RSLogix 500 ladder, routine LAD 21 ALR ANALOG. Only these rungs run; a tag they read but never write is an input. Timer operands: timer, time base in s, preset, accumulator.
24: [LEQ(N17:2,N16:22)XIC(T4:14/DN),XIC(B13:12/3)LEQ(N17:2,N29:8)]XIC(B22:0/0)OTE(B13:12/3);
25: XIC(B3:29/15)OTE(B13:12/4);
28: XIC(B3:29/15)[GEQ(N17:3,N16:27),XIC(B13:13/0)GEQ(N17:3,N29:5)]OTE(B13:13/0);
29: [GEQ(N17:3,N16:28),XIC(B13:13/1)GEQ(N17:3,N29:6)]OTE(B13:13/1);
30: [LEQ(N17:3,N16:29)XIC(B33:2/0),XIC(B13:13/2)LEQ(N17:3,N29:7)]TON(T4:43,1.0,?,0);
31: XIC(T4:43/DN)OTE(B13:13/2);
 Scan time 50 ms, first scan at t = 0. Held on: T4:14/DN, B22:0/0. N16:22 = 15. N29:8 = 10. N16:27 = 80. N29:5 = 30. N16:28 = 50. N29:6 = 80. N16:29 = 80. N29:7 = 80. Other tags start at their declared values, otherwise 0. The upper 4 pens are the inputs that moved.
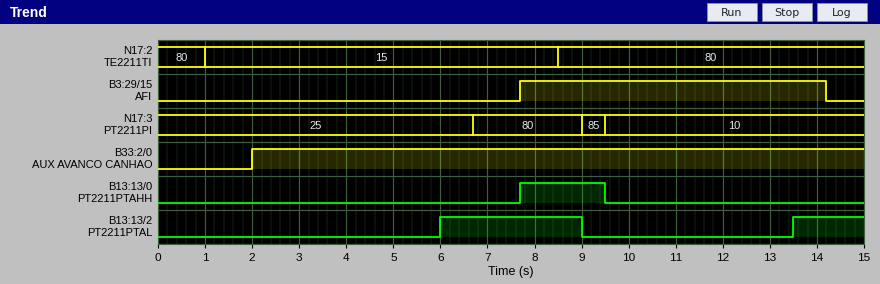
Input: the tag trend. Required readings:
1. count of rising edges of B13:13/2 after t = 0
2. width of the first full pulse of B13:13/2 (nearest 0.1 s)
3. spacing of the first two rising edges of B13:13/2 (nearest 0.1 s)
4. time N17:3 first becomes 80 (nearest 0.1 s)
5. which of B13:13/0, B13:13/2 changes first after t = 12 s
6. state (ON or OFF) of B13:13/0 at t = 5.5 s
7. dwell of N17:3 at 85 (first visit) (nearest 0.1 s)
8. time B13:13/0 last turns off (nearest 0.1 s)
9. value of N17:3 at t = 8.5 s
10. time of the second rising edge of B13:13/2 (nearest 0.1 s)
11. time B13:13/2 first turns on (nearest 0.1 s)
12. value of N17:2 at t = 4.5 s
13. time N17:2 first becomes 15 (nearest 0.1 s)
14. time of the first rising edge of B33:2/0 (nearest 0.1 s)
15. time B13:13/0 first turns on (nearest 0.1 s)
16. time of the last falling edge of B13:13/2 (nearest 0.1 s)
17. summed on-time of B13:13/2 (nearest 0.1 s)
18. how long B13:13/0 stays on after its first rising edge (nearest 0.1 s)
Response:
2
3.0 s
7.5 s
6.7 s
B13:13/2
OFF
0.5 s
9.5 s
80
13.5 s
6.0 s
15
1.0 s
2.0 s
7.7 s
9.0 s
4.5 s
1.8 s
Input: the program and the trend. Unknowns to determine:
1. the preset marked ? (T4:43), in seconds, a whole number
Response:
4 s
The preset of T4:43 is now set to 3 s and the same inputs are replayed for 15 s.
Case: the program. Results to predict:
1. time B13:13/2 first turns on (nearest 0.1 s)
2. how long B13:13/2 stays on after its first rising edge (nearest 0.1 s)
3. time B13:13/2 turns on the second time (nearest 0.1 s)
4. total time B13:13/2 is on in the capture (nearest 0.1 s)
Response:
5.0 s
4.0 s
12.5 s
6.5 s
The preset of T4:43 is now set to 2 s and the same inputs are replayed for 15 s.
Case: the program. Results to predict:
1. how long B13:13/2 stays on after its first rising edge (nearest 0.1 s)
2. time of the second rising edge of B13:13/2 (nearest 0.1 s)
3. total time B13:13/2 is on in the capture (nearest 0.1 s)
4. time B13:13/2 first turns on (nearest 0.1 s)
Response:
5.0 s
11.5 s
8.5 s
4.0 s
